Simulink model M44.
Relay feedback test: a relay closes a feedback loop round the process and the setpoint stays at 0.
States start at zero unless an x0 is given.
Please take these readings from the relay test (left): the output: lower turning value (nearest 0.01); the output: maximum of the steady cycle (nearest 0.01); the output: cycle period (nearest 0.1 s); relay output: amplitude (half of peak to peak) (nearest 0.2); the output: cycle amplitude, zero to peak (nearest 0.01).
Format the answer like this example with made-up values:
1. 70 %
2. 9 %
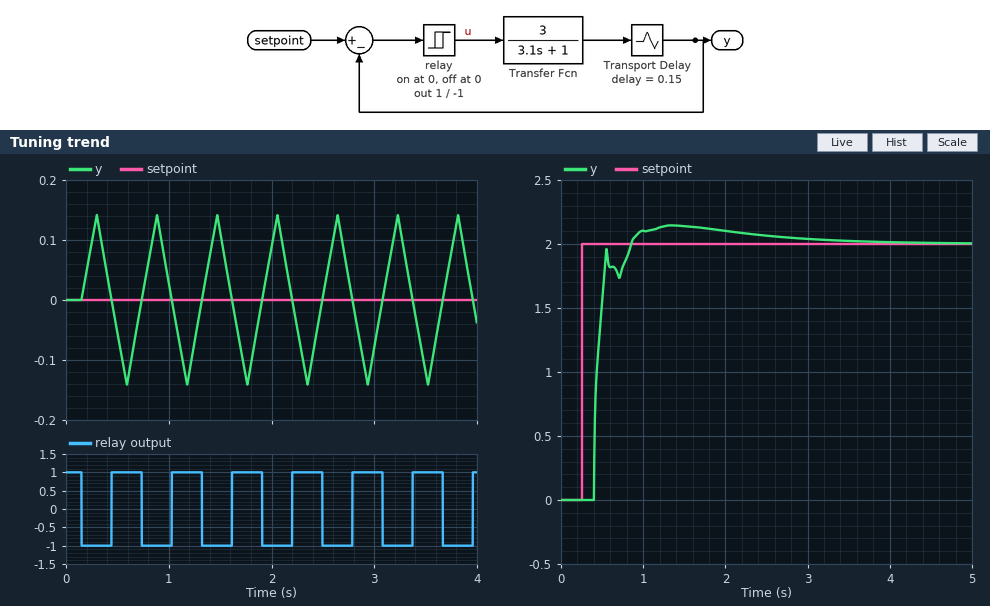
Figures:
1. -0.14
2. 0.14
3. 0.6 s
4. 1.0
5. 0.14
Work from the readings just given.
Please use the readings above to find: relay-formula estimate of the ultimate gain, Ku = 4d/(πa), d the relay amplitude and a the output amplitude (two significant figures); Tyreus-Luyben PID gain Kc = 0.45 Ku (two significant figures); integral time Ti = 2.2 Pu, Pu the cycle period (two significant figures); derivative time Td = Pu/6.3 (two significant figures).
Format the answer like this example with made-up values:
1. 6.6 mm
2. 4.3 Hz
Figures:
1. 9.1
2. 4.1
3. 1.3 s
4. 0.095 s
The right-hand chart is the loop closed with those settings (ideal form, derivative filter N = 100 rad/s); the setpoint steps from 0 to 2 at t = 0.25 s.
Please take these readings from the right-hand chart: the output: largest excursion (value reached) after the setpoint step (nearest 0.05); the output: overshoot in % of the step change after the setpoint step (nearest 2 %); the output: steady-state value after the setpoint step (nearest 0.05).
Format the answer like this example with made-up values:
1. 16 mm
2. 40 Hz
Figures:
1. 2.15
2. 8 %
3. 2.00
